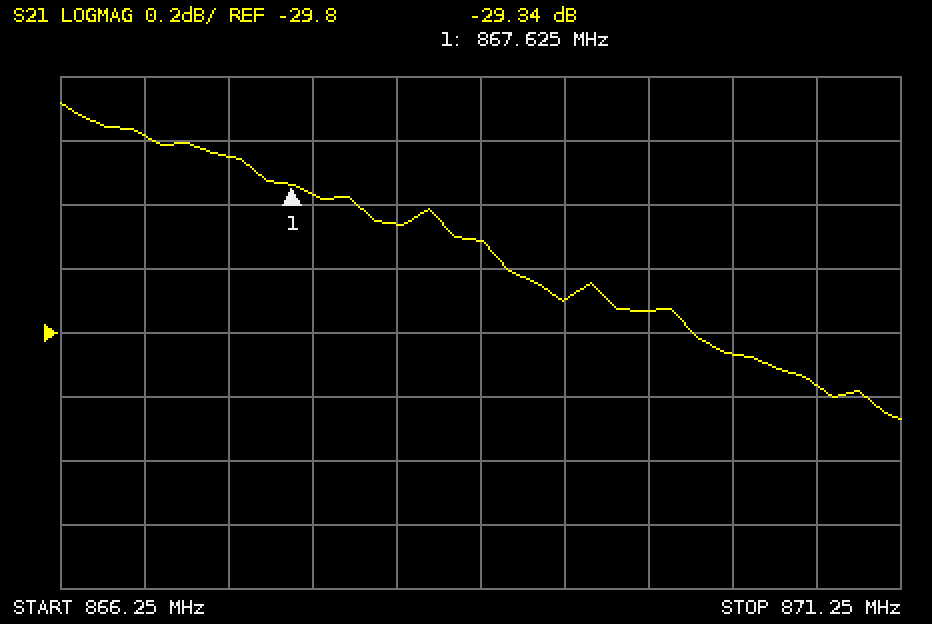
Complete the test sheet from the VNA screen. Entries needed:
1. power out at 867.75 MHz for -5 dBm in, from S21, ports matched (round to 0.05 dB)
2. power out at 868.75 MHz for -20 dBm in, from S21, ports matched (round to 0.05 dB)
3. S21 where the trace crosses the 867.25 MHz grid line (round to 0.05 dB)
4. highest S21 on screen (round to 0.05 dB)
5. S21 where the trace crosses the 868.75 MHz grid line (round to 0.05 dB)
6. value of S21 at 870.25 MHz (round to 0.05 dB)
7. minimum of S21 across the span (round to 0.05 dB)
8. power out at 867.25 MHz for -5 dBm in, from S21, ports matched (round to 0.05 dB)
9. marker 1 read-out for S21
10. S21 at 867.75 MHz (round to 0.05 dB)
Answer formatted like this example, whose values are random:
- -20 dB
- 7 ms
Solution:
- -34.35 dBm
- -49.50 dBm
- -29.25 dB
- -29.10 dB
- -29.50 dB
- -29.85 dB
- -30.05 dB
- -34.25 dBm
- -29.34 dB
- -29.35 dB
